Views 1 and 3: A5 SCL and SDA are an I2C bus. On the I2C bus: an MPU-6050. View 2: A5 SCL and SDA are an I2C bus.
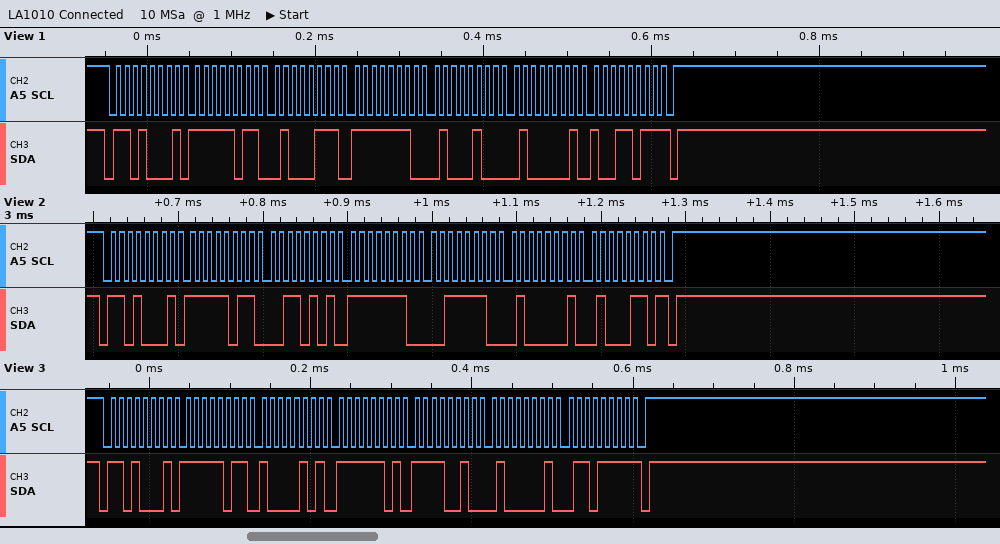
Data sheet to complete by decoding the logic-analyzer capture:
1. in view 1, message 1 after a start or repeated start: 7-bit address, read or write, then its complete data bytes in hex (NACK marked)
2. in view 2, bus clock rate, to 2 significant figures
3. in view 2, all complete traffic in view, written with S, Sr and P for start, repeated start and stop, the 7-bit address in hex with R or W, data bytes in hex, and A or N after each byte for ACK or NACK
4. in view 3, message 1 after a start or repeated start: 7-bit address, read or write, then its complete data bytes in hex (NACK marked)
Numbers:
0x68 read: FB 47 FE 44 41 9B NACK
100 kHz
S 68R A FB A 35 A FE A 3E A 41 A 46 N P
0x68 read: FB 85 FD F2 41 6F NACK
